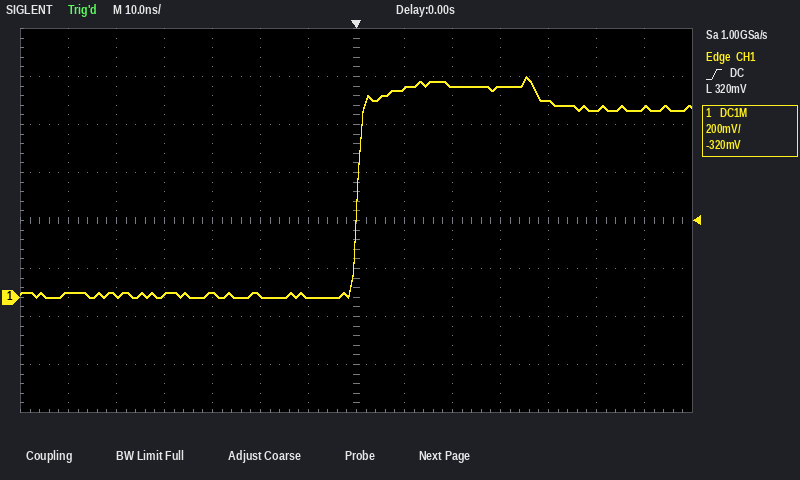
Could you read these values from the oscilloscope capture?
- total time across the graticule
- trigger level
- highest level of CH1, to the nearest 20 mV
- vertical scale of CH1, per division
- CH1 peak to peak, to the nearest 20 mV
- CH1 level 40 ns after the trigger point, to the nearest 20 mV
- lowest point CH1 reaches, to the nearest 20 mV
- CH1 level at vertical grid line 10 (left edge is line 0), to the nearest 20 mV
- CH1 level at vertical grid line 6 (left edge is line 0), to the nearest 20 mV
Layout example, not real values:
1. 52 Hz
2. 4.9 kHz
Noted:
1. 140 ns
2. 320 mV
3. 920 mV
4. 200 mV
5. 920 mV
6. 820 mV
7. 0 mV
8. 880 mV
9. 0 mV
